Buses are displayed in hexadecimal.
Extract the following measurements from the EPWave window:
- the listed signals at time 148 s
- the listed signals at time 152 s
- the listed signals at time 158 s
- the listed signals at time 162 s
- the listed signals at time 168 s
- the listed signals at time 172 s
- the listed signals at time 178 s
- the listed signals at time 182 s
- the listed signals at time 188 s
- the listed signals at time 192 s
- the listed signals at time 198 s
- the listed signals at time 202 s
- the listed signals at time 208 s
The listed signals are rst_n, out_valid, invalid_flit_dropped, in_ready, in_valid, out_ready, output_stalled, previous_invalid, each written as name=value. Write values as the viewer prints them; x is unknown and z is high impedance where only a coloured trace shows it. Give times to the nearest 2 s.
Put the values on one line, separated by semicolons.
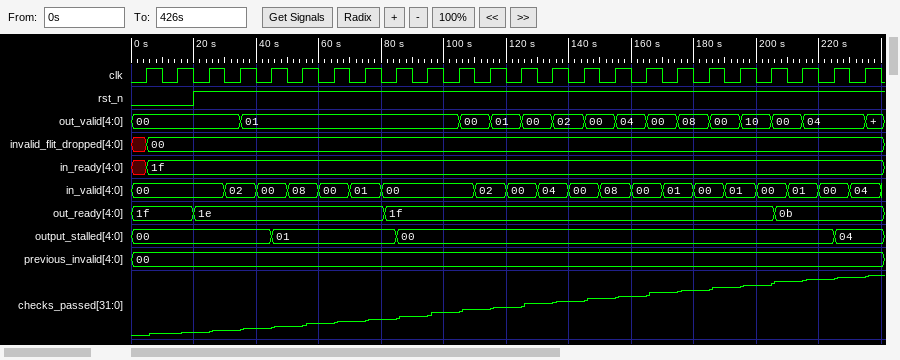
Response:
rst_n=1, out_valid=00, invalid_flit_dropped=00, in_ready=1f, in_valid=00, out_ready=1f, output_stalled=00, previous_invalid=00; rst_n=1, out_valid=00, invalid_flit_dropped=00, in_ready=1f, in_valid=08, out_ready=1f, output_stalled=00, previous_invalid=00; rst_n=1, out_valid=04, invalid_flit_dropped=00, in_ready=1f, in_valid=08, out_ready=1f, output_stalled=00, previous_invalid=00; rst_n=1, out_valid=04, invalid_flit_dropped=00, in_ready=1f, in_valid=00, out_ready=1f, output_stalled=00, previous_invalid=00; rst_n=1, out_valid=00, invalid_flit_dropped=00, in_ready=1f, in_valid=00, out_ready=1f, output_stalled=00, previous_invalid=00; rst_n=1, out_valid=00, invalid_flit_dropped=00, in_ready=1f, in_valid=01, out_ready=1f, output_stalled=00, previous_invalid=00; rst_n=1, out_valid=08, invalid_flit_dropped=00, in_ready=1f, in_valid=01, out_ready=1f, output_stalled=00, previous_invalid=00; rst_n=1, out_valid=08, invalid_flit_dropped=00, in_ready=1f, in_valid=00, out_ready=1f, output_stalled=00, previous_invalid=00; rst_n=1, out_valid=00, invalid_flit_dropped=00, in_ready=1f, in_valid=00, out_ready=1f, output_stalled=00, previous_invalid=00; rst_n=1, out_valid=00, invalid_flit_dropped=00, in_ready=1f, in_valid=01, out_ready=1f, output_stalled=00, previous_invalid=00; rst_n=1, out_valid=10, invalid_flit_dropped=00, in_ready=1f, in_valid=01, out_ready=1f, output_stalled=00, previous_invalid=00; rst_n=1, out_valid=10, invalid_flit_dropped=00, in_ready=1f, in_valid=00, out_ready=1f, output_stalled=00, previous_invalid=00; rst_n=1, out_valid=00, invalid_flit_dropped=00, in_ready=1f, in_valid=00, out_ready=0b, output_stalled=00, previous_invalid=00
